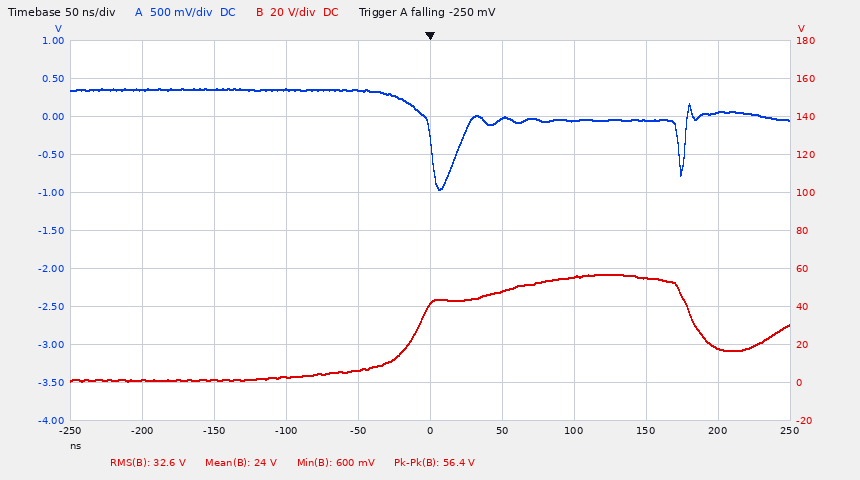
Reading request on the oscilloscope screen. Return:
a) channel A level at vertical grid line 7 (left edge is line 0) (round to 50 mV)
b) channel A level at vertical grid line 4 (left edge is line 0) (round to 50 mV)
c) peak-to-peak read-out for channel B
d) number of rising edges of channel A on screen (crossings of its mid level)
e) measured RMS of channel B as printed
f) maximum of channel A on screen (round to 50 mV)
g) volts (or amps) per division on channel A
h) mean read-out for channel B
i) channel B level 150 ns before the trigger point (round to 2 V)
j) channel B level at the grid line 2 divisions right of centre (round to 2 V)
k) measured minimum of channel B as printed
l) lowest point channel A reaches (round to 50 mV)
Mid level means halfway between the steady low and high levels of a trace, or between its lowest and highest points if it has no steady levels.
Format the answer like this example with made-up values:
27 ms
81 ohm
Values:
-50 mV
350 mV
56.4 V
2
32.6 V
350 mV
500 mV
24 V
2 V
56 V
600 mV
-950 mV
